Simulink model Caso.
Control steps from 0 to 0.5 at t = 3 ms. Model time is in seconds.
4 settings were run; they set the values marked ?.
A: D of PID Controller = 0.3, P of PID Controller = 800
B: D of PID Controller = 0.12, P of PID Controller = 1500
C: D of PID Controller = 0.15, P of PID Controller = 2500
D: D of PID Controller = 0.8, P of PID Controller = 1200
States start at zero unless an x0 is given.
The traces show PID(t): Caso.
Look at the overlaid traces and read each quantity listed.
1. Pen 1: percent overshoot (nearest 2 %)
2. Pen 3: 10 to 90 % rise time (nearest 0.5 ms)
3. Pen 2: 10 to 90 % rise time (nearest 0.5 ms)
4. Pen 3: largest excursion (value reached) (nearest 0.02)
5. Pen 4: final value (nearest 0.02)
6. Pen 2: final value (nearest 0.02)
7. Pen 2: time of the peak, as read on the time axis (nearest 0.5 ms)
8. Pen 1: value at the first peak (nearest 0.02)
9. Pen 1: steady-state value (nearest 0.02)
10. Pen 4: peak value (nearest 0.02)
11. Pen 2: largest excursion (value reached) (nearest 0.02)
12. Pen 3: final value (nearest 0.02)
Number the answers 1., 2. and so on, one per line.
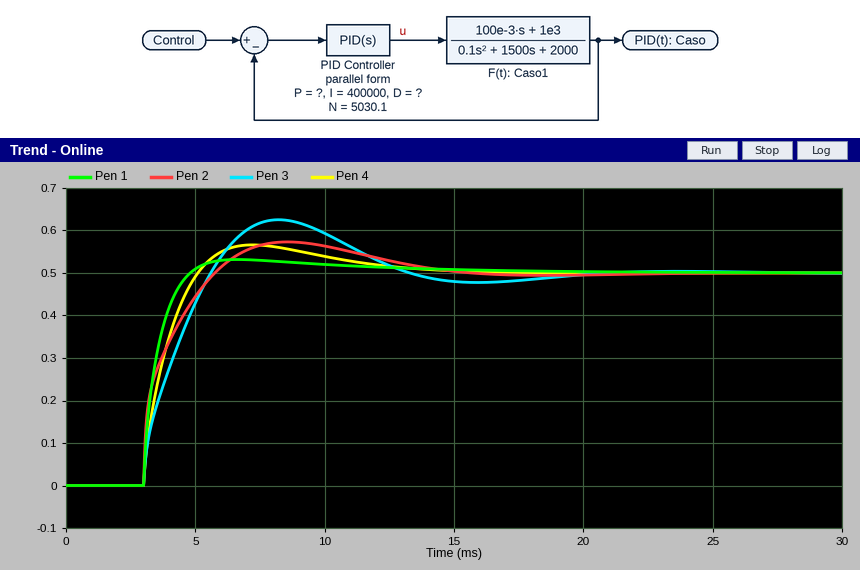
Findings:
1. 6 %
2. 2.0 ms
3. 2.0 ms
4. 0.62
5. 0.50
6. 0.50
7. 8.5 ms
8. 0.54
9. 0.50
10. 0.56
11. 0.58
12. 0.50
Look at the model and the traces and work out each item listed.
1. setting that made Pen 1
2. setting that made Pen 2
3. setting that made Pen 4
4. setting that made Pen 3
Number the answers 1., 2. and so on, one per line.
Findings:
1. C
2. D
3. B
4. A
